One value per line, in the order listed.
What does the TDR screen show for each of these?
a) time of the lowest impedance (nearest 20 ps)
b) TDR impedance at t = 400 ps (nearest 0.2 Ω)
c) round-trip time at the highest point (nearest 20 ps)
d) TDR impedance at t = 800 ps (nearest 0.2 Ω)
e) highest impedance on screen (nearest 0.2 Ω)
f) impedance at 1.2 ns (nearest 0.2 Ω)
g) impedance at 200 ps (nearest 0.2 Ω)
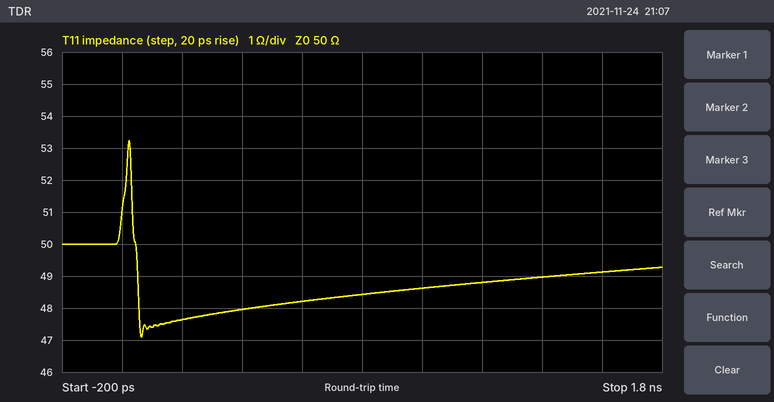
60 ps
48.0 Ω
20 ps
48.4 Ω
53.2 Ω
48.8 Ω
47.6 Ω
